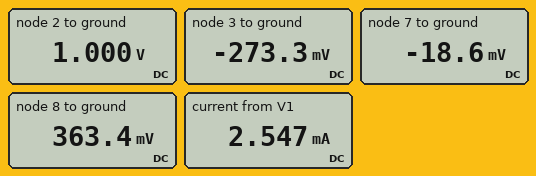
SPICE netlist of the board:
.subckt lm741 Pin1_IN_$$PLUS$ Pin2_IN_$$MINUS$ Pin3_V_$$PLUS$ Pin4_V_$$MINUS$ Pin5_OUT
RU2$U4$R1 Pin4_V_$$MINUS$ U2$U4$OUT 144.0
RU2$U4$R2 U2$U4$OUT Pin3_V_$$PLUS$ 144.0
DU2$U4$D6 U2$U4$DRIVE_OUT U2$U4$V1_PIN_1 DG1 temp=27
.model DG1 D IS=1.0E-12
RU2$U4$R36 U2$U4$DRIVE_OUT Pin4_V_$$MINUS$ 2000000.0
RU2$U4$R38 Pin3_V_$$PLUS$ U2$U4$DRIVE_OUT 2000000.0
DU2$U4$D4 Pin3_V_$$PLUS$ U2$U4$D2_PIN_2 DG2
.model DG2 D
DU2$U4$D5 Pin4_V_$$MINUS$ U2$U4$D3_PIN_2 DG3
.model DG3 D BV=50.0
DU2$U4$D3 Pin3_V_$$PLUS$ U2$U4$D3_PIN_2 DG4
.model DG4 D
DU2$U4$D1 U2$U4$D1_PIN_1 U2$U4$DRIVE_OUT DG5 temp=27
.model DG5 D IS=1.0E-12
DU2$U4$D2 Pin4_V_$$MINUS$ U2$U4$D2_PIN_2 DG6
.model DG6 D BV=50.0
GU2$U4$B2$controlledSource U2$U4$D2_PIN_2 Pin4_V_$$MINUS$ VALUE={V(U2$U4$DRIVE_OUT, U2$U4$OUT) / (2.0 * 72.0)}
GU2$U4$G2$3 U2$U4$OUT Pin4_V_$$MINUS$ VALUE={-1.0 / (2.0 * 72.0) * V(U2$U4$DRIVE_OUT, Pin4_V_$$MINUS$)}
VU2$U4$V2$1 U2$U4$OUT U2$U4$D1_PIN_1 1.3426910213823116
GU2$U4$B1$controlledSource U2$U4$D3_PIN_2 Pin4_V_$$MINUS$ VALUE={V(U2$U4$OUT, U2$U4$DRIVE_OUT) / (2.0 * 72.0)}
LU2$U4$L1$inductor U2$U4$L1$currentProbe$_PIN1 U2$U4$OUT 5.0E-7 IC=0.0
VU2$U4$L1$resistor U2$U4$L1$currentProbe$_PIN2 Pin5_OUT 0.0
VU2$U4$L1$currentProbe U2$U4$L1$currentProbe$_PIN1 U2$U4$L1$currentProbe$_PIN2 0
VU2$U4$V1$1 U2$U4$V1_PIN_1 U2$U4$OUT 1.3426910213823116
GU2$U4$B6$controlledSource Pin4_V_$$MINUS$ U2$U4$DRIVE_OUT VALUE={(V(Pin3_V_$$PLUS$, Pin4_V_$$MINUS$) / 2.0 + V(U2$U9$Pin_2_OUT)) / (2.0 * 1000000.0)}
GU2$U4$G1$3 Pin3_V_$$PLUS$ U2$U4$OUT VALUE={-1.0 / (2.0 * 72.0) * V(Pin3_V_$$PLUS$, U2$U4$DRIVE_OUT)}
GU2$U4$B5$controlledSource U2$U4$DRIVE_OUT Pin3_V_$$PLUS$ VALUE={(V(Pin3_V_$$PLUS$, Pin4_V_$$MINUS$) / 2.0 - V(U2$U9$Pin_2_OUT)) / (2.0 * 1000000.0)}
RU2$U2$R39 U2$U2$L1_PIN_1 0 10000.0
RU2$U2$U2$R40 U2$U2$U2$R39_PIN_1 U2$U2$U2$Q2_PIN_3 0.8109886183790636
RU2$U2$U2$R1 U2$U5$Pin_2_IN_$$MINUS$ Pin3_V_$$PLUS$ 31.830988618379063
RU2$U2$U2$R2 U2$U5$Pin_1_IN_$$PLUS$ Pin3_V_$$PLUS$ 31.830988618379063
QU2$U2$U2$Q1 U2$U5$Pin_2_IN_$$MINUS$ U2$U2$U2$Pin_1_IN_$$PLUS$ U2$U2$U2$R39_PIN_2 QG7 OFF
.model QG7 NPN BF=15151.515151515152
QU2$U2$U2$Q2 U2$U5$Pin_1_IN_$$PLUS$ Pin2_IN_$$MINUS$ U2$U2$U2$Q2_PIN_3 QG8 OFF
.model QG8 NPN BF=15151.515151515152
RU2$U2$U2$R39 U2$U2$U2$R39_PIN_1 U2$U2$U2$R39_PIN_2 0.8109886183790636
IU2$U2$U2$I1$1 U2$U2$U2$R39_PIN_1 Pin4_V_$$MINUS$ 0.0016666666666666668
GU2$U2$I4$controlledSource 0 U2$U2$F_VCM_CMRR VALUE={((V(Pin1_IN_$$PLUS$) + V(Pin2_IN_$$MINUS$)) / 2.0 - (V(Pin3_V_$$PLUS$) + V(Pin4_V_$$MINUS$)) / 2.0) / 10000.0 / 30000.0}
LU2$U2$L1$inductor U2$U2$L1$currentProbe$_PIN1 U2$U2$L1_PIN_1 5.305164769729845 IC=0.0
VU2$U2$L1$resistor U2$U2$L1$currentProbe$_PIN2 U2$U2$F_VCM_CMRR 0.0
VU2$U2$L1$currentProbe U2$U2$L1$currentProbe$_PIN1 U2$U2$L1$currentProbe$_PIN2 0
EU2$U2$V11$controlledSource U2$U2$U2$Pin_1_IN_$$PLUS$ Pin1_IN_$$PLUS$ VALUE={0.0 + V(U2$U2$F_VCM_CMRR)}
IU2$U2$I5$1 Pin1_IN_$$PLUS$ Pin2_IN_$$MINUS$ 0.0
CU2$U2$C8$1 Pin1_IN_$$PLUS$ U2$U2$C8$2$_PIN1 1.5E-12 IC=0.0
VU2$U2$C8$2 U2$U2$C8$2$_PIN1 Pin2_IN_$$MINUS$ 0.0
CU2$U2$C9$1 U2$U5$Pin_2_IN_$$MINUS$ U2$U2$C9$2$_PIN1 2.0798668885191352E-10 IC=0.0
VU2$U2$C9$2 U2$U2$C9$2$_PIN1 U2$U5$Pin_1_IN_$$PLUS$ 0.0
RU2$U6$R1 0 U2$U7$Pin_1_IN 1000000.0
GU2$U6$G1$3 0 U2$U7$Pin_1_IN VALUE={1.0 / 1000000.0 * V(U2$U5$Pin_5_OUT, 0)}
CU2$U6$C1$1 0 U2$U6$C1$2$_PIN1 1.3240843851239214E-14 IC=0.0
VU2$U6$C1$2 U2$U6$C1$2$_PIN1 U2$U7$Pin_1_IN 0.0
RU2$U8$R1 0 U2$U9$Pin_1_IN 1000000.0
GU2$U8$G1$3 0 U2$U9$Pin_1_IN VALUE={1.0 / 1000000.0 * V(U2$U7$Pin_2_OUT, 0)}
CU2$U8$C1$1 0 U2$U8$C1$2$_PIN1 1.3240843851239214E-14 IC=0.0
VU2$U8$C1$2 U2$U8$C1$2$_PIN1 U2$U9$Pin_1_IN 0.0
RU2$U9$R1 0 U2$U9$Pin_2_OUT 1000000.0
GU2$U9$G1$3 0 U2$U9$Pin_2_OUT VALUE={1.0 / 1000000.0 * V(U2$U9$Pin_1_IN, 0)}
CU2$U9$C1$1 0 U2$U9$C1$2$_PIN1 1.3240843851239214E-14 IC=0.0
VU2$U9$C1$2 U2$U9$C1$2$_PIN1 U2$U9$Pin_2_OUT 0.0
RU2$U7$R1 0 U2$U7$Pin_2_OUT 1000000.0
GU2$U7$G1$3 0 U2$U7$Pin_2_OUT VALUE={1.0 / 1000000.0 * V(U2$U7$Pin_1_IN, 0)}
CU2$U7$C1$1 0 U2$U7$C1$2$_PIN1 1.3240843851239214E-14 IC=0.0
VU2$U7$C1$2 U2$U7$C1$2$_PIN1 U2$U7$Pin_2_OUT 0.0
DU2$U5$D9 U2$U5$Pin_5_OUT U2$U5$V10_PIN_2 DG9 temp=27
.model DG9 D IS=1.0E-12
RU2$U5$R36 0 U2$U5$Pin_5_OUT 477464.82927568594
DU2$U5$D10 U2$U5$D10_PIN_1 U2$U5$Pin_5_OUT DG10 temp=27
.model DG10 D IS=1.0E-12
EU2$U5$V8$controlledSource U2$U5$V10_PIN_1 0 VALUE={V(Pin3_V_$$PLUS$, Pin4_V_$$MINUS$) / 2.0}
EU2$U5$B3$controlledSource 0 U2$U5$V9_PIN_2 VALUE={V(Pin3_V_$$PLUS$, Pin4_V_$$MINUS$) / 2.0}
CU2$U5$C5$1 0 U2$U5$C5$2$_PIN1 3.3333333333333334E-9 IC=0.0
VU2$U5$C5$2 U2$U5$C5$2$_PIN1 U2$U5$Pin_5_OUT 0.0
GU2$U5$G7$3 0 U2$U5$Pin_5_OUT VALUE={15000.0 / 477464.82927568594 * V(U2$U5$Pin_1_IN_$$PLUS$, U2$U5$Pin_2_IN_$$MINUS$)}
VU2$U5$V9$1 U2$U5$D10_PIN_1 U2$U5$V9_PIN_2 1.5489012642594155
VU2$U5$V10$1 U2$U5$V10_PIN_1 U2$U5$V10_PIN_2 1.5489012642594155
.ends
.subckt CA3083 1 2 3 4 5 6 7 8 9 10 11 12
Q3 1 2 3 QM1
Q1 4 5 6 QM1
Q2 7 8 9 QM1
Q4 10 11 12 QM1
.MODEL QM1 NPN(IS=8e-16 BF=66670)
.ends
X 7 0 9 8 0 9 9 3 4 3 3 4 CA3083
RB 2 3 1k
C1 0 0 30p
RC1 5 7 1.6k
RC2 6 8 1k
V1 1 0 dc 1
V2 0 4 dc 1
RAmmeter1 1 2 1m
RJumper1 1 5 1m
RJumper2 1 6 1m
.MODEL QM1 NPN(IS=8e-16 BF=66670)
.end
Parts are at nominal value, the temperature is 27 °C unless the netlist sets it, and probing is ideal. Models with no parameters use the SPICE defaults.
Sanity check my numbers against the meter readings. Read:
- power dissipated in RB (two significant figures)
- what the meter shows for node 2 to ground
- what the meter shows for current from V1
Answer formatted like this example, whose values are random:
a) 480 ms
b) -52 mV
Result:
a) 1.6 mW
b) 1.000 V
c) 2.547 mA
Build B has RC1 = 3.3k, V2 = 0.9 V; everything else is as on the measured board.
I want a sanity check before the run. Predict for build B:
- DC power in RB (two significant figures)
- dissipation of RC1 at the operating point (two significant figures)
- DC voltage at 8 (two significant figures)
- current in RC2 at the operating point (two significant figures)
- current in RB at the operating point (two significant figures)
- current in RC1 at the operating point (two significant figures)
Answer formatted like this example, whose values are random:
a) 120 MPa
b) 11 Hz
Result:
a) 1.4 mW
b) 820 µW
c) 380 mV
d) 620 µA
e) 1.2 mA
f) 500 µA
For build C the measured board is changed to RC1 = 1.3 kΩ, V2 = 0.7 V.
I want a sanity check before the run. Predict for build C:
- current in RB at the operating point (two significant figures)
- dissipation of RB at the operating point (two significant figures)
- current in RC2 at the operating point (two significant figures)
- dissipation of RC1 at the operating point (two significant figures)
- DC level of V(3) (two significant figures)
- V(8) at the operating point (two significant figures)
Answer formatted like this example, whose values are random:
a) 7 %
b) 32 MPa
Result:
a) 990 µA
b) 970 µW
c) 140 µA
d) 26 µW
e) 13 mV
f) 860 mV
